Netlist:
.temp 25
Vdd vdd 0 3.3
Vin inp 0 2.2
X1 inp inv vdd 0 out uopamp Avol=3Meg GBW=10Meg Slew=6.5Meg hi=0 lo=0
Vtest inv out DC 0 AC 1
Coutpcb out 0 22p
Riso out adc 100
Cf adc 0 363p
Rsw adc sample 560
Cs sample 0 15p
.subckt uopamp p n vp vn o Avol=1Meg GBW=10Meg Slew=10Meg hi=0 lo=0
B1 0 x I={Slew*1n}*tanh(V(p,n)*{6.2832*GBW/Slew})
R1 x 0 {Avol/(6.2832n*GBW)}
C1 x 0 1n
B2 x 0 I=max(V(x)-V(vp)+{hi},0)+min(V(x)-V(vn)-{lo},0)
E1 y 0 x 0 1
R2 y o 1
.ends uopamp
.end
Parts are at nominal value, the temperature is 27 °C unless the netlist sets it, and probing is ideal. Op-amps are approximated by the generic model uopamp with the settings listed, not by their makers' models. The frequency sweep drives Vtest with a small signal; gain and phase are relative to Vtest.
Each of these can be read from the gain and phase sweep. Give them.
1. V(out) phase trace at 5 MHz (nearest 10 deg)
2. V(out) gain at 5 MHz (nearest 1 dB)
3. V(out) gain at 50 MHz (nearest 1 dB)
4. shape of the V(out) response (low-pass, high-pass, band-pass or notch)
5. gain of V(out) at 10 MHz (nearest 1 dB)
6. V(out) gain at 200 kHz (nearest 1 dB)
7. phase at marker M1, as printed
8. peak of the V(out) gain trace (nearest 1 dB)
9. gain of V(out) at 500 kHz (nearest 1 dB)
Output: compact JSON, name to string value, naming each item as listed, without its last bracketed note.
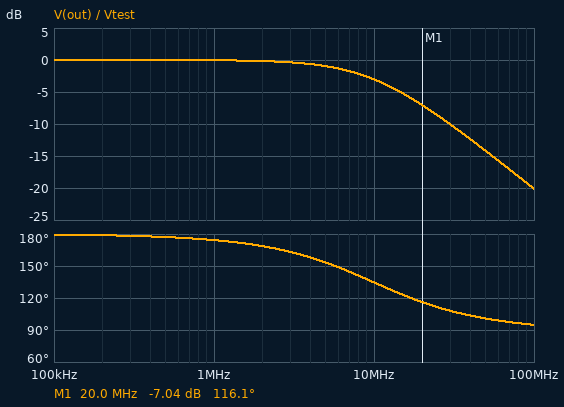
{"V(out) phase trace at 5 MHz": "150 deg", "V(out) gain at 5 MHz": "-1 dB", "V(out) gain at 50 MHz": "-14 dB", "shape of the V(out) response": "low-pass", "gain of V(out) at 10 MHz": "-3 dB", "V(out) gain at 200 kHz": "0 dB", "phase at marker M1, as printed": "116.1 deg", "peak of the V(out) gain trace": "0 dB", "gain of V(out) at 500 kHz": "0 dB"}
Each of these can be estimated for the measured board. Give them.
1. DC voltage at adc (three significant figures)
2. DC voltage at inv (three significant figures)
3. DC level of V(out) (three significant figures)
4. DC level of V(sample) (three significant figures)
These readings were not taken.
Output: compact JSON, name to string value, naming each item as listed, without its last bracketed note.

{"DC voltage at adc": "2.20 V", "DC voltage at inv": "2.20 V", "DC level of V(out)": "2.20 V", "DC level of V(sample)": "2.20 V"}
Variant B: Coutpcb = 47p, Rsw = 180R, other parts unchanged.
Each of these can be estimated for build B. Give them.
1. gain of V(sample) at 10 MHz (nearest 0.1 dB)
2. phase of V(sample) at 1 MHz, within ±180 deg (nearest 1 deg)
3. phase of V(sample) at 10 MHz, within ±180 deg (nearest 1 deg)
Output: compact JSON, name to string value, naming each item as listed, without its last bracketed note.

{"gain of V(sample) at 10 MHz": "-11.4 dB", "phase of V(sample) at 1 MHz, within ±180 deg": "160 deg", "phase of V(sample) at 10 MHz, within ±180 deg": "58 deg"}
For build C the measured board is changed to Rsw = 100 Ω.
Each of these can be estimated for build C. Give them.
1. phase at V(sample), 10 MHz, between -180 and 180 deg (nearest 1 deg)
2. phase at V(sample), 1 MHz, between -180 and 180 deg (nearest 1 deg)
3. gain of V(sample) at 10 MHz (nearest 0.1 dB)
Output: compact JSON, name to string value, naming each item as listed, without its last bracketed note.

{"phase at V(sample), 10 MHz, between -180 and 180 deg": "62 deg", "phase at V(sample), 1 MHz, between -180 and 180 deg": "160 deg", "gain of V(sample) at 10 MHz": "-11.3 dB"}
